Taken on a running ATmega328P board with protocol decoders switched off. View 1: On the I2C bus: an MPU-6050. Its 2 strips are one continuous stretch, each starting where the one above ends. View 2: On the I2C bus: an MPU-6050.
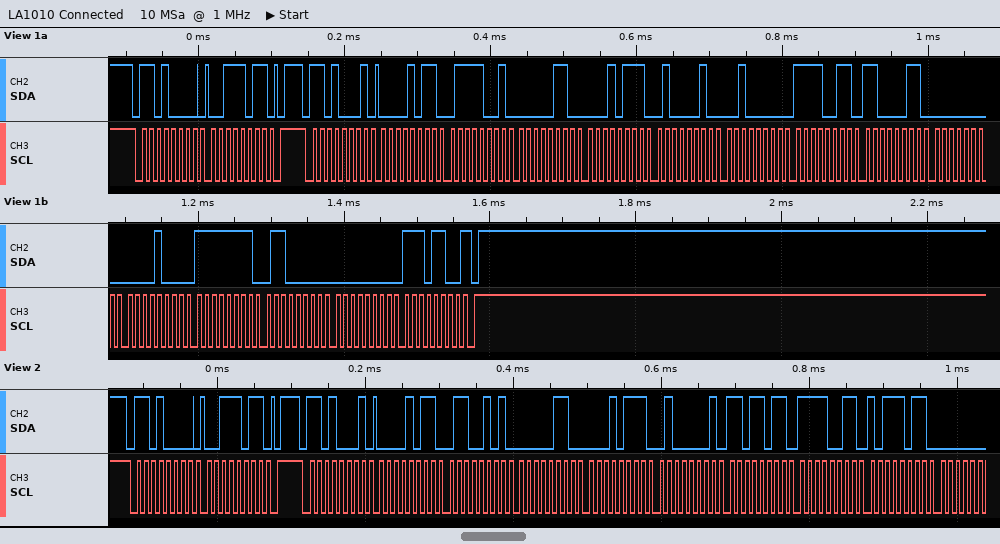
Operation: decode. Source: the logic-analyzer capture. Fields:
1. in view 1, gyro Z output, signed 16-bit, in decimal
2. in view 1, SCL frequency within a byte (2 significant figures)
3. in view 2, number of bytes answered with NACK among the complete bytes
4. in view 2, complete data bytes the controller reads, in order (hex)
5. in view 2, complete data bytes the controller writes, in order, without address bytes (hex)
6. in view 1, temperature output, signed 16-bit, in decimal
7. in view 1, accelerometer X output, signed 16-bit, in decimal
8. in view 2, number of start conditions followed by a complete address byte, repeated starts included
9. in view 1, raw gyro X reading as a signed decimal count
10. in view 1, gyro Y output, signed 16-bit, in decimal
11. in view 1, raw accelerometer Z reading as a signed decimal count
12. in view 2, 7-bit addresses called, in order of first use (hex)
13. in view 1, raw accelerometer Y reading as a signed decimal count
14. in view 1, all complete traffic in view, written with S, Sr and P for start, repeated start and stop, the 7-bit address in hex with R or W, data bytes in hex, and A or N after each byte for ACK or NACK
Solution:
236
100 kHz
0
0B 65 06 17 41 DB F3 BB
3B
-3133
2937
2
8
-160
16928
0x68
1559
S 68W A 3B A P S 68R A 0B A 79 A 06 A 17 A 42 A 20 A F3 A C3 A 00 A 08 A FF A 60 A 00 A EC N P
